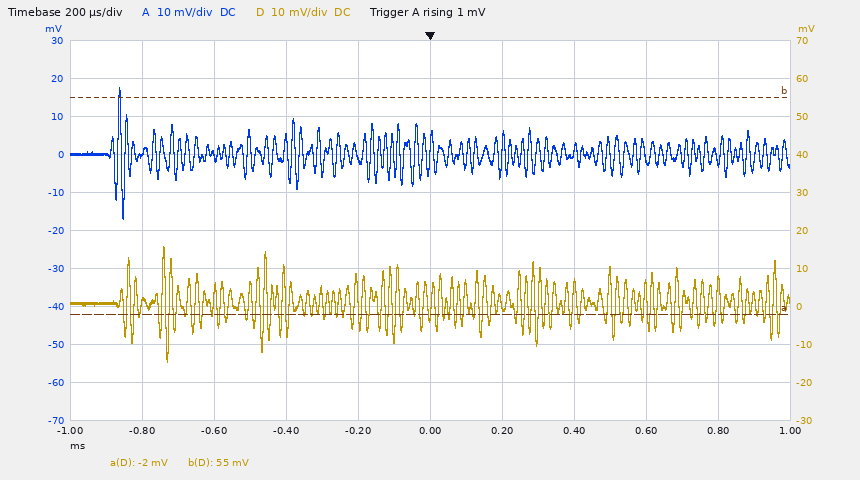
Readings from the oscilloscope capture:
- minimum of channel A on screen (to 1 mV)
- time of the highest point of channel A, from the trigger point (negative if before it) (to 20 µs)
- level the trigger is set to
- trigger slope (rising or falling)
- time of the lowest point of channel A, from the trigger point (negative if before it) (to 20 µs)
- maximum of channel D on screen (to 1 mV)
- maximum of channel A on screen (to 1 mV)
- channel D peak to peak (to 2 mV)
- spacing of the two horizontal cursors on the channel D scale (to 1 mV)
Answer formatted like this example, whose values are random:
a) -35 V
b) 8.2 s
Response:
a) -17 mV
b) -860 µs
c) 1 mV
d) rising
e) -860 µs
f) 16 mV
g) 18 mV
h) 30 mV
i) 57 mV
